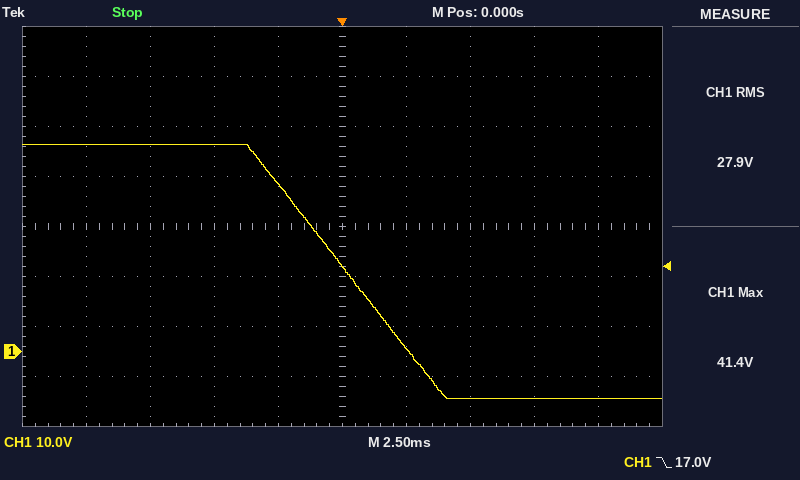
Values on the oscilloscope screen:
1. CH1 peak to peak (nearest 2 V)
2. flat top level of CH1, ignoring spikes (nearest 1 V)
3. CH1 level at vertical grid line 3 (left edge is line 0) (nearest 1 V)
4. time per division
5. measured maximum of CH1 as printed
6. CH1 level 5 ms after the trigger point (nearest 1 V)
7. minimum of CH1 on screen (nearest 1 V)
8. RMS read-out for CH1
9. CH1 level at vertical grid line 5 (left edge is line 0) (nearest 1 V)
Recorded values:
50 V
41 V
41 V
2.5 ms
41.4 V
-9 V
-9 V
27.9 V
17 V
